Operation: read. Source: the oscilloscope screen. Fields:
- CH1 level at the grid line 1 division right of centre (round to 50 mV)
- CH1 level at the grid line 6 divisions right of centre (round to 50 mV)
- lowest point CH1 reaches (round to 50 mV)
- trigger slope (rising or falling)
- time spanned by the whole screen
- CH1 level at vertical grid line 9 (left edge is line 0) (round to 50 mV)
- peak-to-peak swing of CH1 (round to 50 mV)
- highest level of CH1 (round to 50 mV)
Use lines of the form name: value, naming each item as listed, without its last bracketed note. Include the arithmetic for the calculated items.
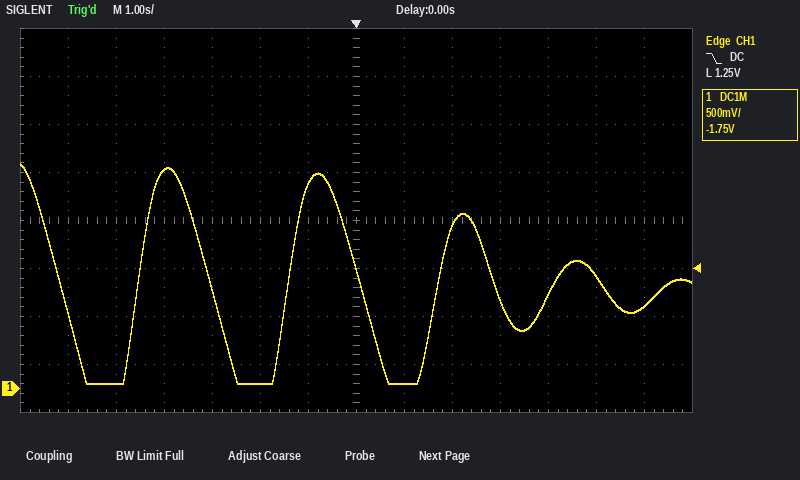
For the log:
CH1 level at the grid line 1 division right of centre: 50 mV
CH1 level at the grid line 6 divisions right of centre: 850 mV
lowest point CH1 reaches: 50 mV
trigger slope: falling
time spanned by the whole screen: 14 s
CH1 level at vertical grid line 9 (left edge is line 0): 1.70 V
peak-to-peak swing of CH1: 2.35 V − (50 mV) = 2.30 V
highest level of CH1: 2.35 V
